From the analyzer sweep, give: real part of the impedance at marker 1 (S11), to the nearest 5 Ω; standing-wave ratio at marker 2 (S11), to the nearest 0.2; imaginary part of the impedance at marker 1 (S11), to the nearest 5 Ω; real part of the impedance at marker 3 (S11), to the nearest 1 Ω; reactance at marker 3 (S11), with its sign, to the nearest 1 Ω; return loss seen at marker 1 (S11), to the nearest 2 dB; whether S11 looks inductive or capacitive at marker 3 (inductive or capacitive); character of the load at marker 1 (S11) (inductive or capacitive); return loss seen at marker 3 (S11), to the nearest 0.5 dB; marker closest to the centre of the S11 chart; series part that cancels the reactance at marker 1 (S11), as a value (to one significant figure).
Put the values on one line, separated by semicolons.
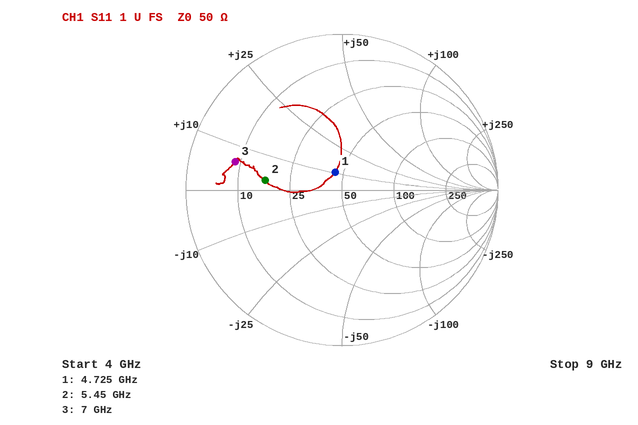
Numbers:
45 Ω; 3.0; +10 Ω; 9 Ω; +6 Ω; 18 dB; inductive; inductive; 3.0 dB; marker 1; 3 pF
